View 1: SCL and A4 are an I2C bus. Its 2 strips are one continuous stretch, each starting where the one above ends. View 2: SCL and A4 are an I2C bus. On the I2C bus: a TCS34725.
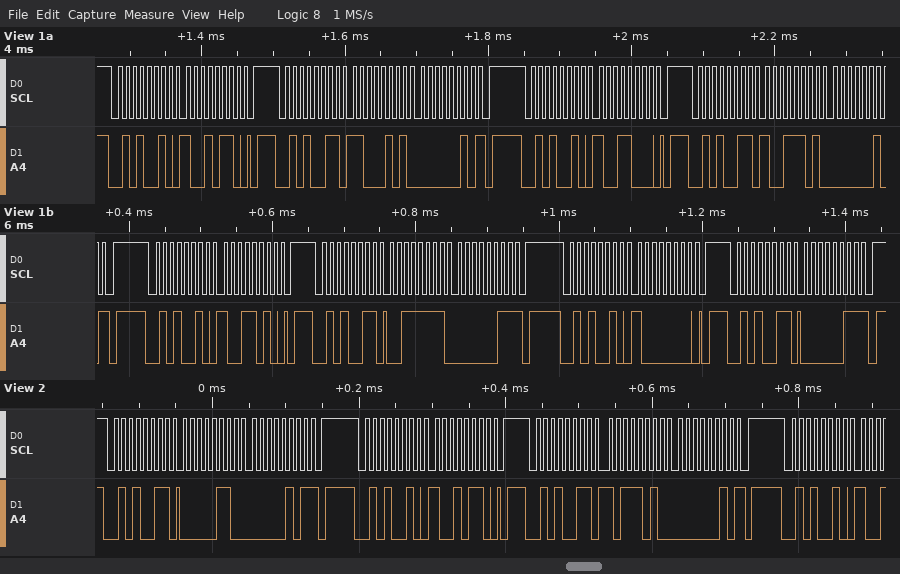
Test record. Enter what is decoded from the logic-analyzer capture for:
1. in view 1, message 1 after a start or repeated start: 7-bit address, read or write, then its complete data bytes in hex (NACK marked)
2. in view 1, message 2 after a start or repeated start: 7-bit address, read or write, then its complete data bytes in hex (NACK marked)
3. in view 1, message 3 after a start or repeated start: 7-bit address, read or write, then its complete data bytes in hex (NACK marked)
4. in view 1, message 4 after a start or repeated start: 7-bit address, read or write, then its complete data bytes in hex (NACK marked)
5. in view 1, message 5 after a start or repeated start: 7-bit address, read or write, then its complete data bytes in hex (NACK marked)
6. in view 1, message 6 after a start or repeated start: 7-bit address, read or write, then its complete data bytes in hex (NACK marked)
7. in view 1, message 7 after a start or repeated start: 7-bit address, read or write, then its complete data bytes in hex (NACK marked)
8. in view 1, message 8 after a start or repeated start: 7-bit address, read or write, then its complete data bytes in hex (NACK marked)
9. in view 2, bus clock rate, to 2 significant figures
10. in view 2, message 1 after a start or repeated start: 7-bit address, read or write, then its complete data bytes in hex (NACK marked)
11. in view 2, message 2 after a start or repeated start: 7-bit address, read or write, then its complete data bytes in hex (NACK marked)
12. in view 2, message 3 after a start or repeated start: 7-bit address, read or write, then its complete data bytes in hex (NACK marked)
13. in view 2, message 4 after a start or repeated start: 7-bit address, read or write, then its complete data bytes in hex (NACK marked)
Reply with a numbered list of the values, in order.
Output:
1. 0x29 write: 96
2. 0x29 read: C5 02 NACK
3. 0x29 write: 98
4. 0x29 read: 9D 02 NACK
5. 0x29 write: 9A
6. 0x29 read: 3F 03 NACK
7. 0x29 write: 80
8. 0x29 read: 03 NACK
9. 100 kHz
10. 0x29 read: 06 05 NACK
11. 0x29 write: 96
12. 0x29 read: BA 02 NACK
13. 0x29 write
